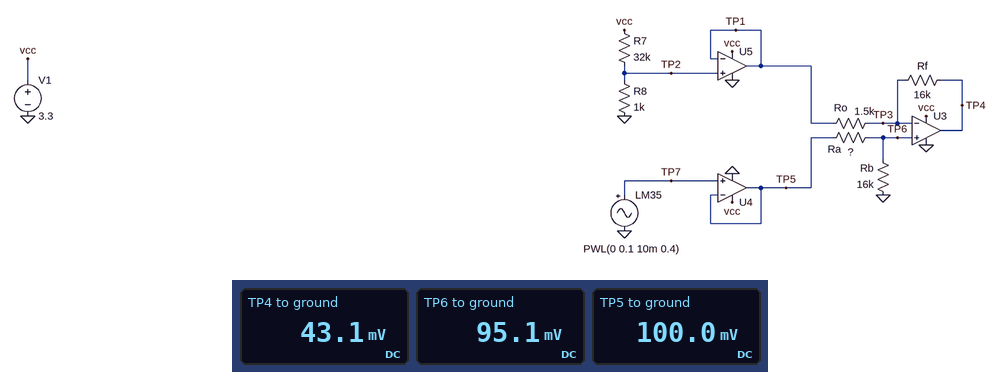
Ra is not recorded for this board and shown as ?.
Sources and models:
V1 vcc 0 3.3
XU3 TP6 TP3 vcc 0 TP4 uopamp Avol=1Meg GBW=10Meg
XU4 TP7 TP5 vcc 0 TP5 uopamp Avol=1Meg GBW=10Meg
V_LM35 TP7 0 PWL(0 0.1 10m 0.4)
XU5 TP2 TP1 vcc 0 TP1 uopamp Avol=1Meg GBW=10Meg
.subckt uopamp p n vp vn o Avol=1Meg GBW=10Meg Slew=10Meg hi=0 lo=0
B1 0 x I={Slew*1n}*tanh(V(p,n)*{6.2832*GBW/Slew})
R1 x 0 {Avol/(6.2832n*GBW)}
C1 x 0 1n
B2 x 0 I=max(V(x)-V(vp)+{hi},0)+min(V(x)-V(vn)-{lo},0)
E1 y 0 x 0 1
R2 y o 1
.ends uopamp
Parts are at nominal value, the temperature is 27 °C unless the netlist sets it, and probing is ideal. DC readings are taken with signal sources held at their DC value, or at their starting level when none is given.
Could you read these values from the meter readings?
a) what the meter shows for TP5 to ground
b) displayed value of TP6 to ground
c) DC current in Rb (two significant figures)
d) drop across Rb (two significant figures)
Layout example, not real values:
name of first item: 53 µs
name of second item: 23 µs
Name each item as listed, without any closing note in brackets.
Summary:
what the meter shows for TP5 to ground: 100.0 mV
displayed value of TP6 to ground: 95.1 mV
DC current in Rb: 5.9 µA
drop across Rb: 95 mV
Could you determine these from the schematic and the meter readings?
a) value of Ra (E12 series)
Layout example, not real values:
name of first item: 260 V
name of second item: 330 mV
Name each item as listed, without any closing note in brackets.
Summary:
value of Ra: 820 Ω
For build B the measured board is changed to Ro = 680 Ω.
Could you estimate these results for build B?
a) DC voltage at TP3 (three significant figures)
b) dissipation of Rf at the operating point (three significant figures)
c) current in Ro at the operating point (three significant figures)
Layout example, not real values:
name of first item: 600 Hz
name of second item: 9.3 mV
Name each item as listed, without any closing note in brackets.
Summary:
DC voltage at TP3: 95.9 mV
dissipation of Rf at the operating point: 576 nW
current in Ro at the operating point: 6.00 µA
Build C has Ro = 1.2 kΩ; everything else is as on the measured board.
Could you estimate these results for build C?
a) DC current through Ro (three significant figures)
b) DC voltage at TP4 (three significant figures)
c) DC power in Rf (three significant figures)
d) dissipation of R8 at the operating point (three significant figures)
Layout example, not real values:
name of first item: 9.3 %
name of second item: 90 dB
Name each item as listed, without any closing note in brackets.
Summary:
DC current through Ro: 4.06 µA
DC voltage at TP4: 30.1 mV
DC power in Rf: 264 nW
dissipation of R8 at the operating point: 10.0 µW
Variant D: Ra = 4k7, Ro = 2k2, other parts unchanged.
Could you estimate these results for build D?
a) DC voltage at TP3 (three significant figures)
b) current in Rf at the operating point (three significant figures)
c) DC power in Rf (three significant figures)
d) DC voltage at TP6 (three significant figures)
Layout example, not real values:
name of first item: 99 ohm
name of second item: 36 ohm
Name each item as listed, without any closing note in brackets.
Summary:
DC voltage at TP3: 87.8 mV
current in Rf at the operating point: 5.53 µA
DC power in Rf: 489 nW
DC voltage at TP6: 77.3 mV
